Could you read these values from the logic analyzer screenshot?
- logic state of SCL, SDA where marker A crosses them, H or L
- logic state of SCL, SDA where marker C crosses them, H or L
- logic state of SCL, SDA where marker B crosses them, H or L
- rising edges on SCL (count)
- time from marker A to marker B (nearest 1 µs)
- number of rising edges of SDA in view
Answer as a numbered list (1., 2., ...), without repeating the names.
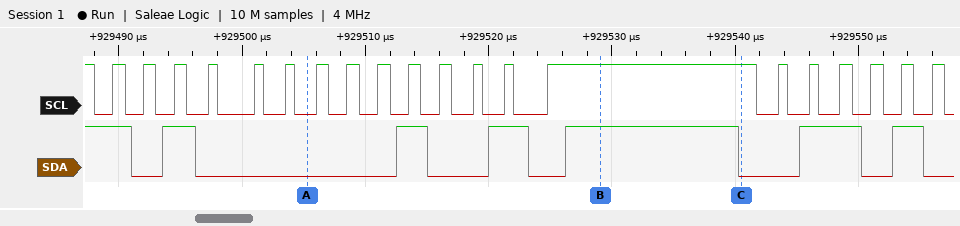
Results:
1. SCL=L, SDA=L
2. SCL=H, SDA=L
3. SCL=H, SDA=H
4. 20
5. 24 µs
6. 6
